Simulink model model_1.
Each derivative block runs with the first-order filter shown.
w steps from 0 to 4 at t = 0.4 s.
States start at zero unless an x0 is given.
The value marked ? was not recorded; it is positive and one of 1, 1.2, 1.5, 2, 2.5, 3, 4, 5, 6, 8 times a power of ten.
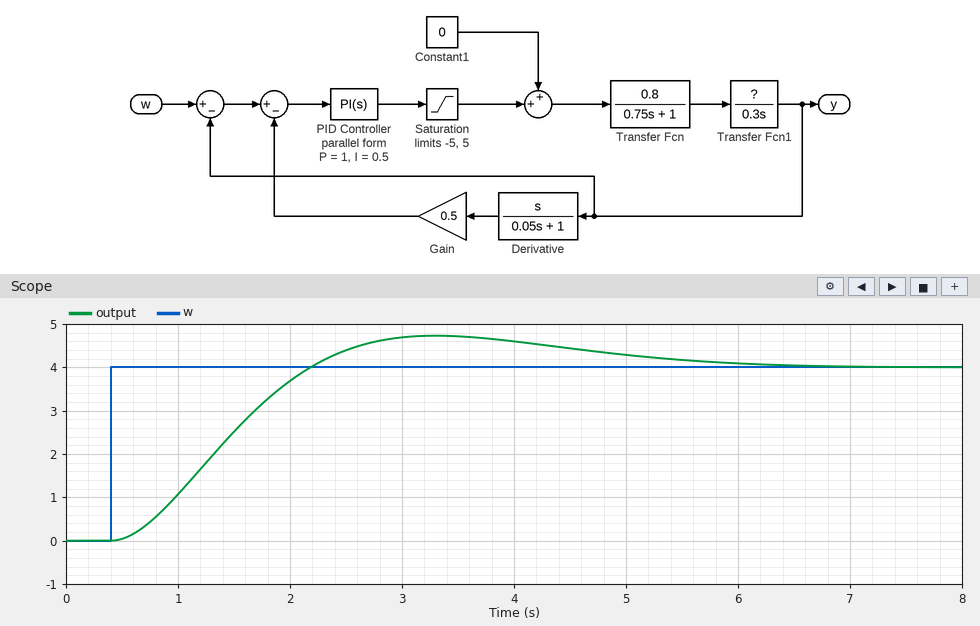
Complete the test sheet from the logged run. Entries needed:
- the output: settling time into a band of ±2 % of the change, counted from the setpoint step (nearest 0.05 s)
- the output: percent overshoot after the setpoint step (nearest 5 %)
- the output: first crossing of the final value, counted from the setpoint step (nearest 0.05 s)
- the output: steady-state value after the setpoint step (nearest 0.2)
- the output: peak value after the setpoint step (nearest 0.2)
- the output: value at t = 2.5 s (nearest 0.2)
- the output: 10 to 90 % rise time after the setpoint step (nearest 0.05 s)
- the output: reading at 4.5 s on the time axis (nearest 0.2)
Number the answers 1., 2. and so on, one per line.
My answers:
1. 5.70 s
2. 20 %
3. 1.80 s
4. 4.0
5. 4.8
6. 4.4
7. 1.20 s
8. 4.4
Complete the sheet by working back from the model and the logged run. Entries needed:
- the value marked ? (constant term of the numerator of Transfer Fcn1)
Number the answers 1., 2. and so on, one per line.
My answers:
1. 0.6
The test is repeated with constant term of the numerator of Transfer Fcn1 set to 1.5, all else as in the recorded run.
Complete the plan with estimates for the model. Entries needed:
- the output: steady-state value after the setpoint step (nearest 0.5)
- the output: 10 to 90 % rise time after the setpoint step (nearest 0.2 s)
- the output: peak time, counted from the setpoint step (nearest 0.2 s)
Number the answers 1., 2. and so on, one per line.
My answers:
1. 4.0
2. 1.0 s
3. 2.2 s
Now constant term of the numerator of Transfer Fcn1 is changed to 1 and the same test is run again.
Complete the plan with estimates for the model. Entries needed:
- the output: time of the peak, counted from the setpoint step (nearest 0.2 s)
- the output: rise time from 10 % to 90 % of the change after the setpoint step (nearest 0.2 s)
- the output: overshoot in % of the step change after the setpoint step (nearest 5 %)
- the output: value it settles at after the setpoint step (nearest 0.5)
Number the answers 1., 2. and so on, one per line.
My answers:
1. 2.4 s
2. 1.0 s
3. 10 %
4. 4.0
